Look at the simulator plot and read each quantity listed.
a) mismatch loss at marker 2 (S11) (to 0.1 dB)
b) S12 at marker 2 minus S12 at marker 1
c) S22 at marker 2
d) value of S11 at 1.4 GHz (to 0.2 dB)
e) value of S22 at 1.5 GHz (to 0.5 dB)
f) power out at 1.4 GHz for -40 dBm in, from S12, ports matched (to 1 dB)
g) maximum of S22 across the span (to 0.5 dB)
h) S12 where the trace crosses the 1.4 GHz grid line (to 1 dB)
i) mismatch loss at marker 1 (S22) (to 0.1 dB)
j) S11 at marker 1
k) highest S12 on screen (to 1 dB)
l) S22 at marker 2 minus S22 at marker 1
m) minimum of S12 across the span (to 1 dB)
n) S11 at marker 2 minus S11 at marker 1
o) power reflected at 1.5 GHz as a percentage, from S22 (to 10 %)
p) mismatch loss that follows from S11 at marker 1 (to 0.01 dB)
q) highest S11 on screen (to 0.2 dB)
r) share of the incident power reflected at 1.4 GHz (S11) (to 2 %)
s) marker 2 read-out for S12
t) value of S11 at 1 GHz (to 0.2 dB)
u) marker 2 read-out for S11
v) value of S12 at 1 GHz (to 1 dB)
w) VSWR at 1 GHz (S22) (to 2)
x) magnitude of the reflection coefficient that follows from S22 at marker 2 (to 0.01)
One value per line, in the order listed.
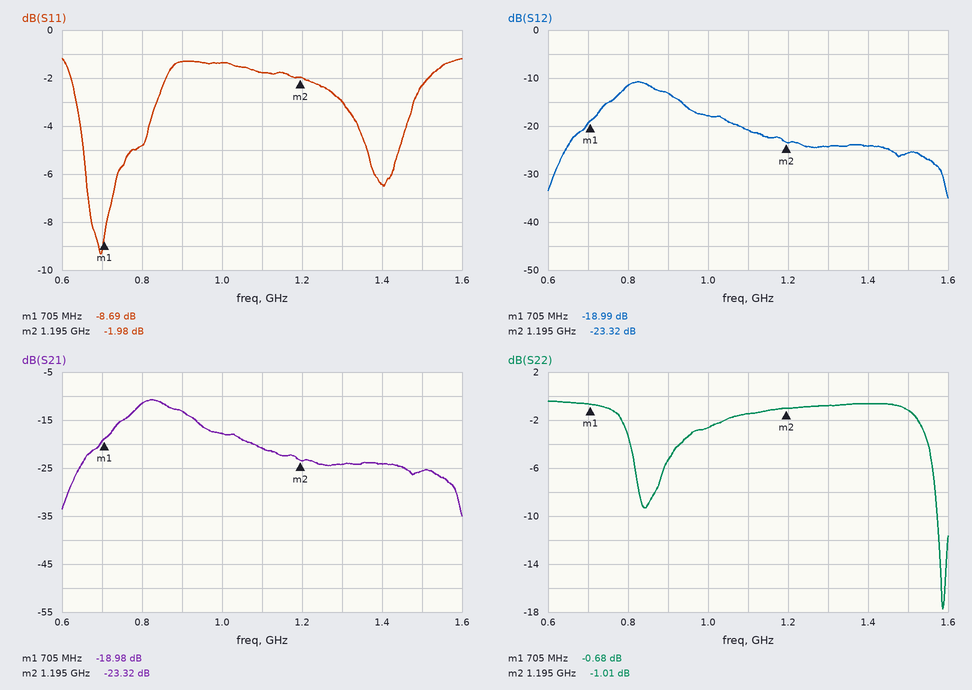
4.4 dB
-4.33 dB
-1.01 dB
-6.4 dB
-1.0 dB
-64 dBm
-0.5 dB
-24 dB
8.4 dB
-8.69 dB
-11 dB
-0.33 dB
-35 dB
6.71 dB
80 %
0.63 dB
-1.2 dB
22 %
-23.32 dB
-1.4 dB
-1.98 dB
-18 dB
6
0.89
